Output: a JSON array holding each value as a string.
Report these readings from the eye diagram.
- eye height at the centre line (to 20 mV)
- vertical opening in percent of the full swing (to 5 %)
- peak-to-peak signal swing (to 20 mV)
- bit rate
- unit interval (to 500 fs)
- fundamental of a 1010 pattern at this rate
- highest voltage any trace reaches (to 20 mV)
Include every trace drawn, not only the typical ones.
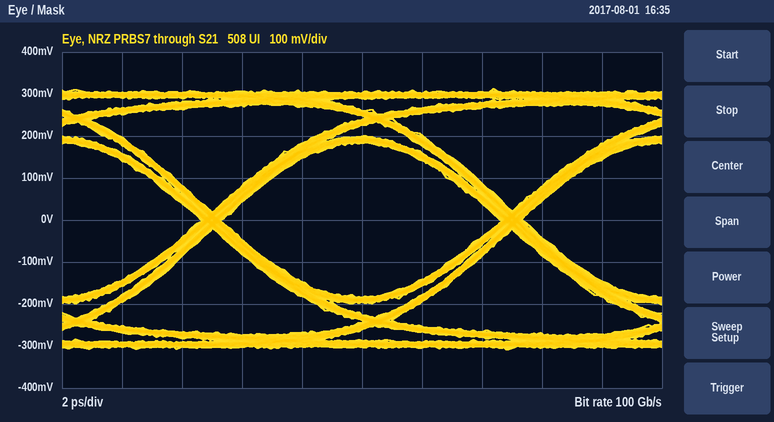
["360 mV", "60 %", "620 mV", "100 Gb/s", "10.0 ps", "50 GHz", "320 mV"]
